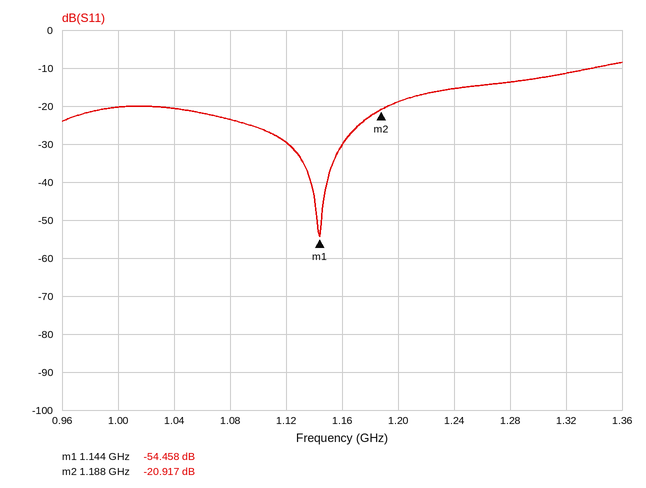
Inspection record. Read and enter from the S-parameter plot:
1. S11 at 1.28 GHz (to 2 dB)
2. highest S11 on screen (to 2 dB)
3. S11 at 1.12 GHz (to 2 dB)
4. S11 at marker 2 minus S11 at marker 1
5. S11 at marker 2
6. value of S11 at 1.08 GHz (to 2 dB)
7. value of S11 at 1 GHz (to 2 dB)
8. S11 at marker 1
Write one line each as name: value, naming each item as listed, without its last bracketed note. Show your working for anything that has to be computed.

S11 at 1.28 GHz: -14 dB
highest S11 on screen: -8 dB
S11 at 1.12 GHz: -30 dB
S11 at marker 2 minus S11 at marker 1: -20.917 − (-54.458) = 33.541 dB
S11 at marker 2: -20.917 dB
value of S11 at 1.08 GHz: -24 dB
value of S11 at 1 GHz: -20 dB
S11 at marker 1: -54.458 dB
